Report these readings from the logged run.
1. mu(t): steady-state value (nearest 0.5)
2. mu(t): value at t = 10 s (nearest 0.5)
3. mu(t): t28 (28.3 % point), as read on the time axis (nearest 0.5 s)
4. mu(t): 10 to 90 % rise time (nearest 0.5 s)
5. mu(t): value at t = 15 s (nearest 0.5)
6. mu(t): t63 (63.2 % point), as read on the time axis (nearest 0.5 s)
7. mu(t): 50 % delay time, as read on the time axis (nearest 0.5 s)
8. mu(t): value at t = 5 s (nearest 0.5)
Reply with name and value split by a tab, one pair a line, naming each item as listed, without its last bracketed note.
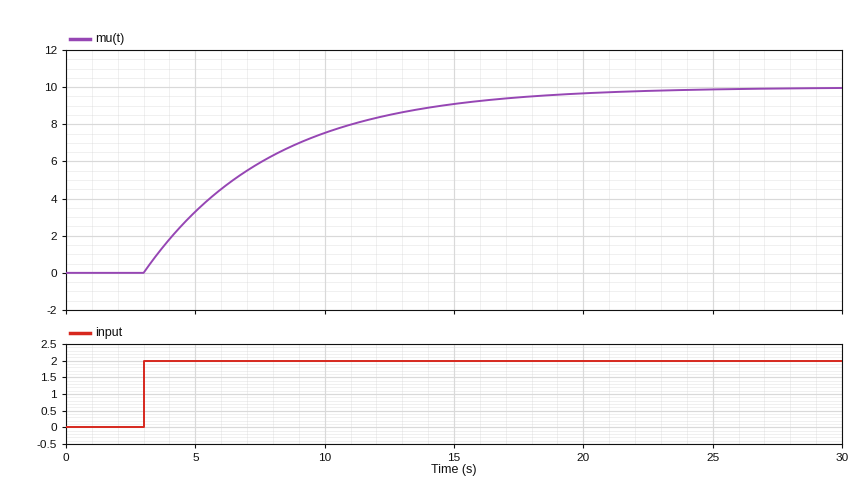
mu(t): steady-state value	10.0
mu(t): value at t = 10 s	7.5
mu(t): t28 (28.3 % point), as read on the time axis	4.5 s
mu(t): 10 to 90 % rise time	11.0 s
mu(t): value at t = 15 s	9.0
mu(t): t63 (63.2 % point), as read on the time axis	8.0 s
mu(t): 50 % delay time, as read on the time axis	6.5 s
mu(t): value at t = 5 s	3.5
